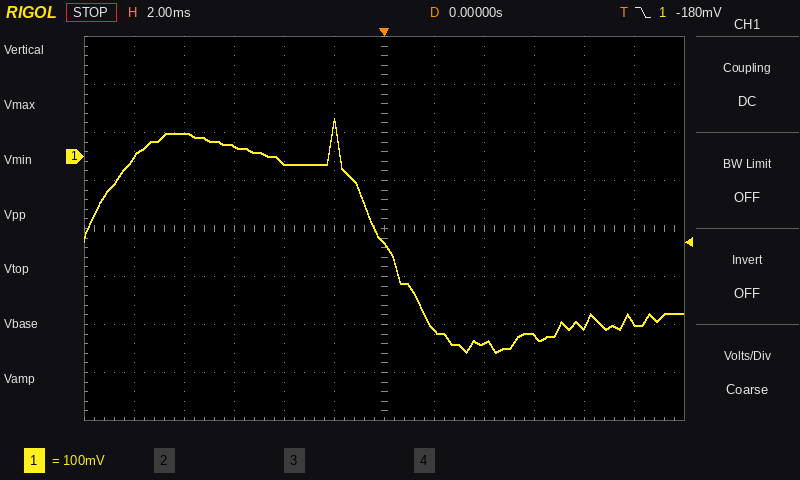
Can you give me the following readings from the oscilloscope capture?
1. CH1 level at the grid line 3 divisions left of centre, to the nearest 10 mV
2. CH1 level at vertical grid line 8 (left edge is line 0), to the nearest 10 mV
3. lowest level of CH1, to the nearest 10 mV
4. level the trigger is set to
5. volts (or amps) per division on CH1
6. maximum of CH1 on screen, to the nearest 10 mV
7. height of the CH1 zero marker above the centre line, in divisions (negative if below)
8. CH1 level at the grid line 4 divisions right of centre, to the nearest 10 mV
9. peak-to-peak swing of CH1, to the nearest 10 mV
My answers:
20 mV
-390 mV
-410 mV
-180 mV
100 mV
80 mV
+1.5 div
-350 mV
490 mV
